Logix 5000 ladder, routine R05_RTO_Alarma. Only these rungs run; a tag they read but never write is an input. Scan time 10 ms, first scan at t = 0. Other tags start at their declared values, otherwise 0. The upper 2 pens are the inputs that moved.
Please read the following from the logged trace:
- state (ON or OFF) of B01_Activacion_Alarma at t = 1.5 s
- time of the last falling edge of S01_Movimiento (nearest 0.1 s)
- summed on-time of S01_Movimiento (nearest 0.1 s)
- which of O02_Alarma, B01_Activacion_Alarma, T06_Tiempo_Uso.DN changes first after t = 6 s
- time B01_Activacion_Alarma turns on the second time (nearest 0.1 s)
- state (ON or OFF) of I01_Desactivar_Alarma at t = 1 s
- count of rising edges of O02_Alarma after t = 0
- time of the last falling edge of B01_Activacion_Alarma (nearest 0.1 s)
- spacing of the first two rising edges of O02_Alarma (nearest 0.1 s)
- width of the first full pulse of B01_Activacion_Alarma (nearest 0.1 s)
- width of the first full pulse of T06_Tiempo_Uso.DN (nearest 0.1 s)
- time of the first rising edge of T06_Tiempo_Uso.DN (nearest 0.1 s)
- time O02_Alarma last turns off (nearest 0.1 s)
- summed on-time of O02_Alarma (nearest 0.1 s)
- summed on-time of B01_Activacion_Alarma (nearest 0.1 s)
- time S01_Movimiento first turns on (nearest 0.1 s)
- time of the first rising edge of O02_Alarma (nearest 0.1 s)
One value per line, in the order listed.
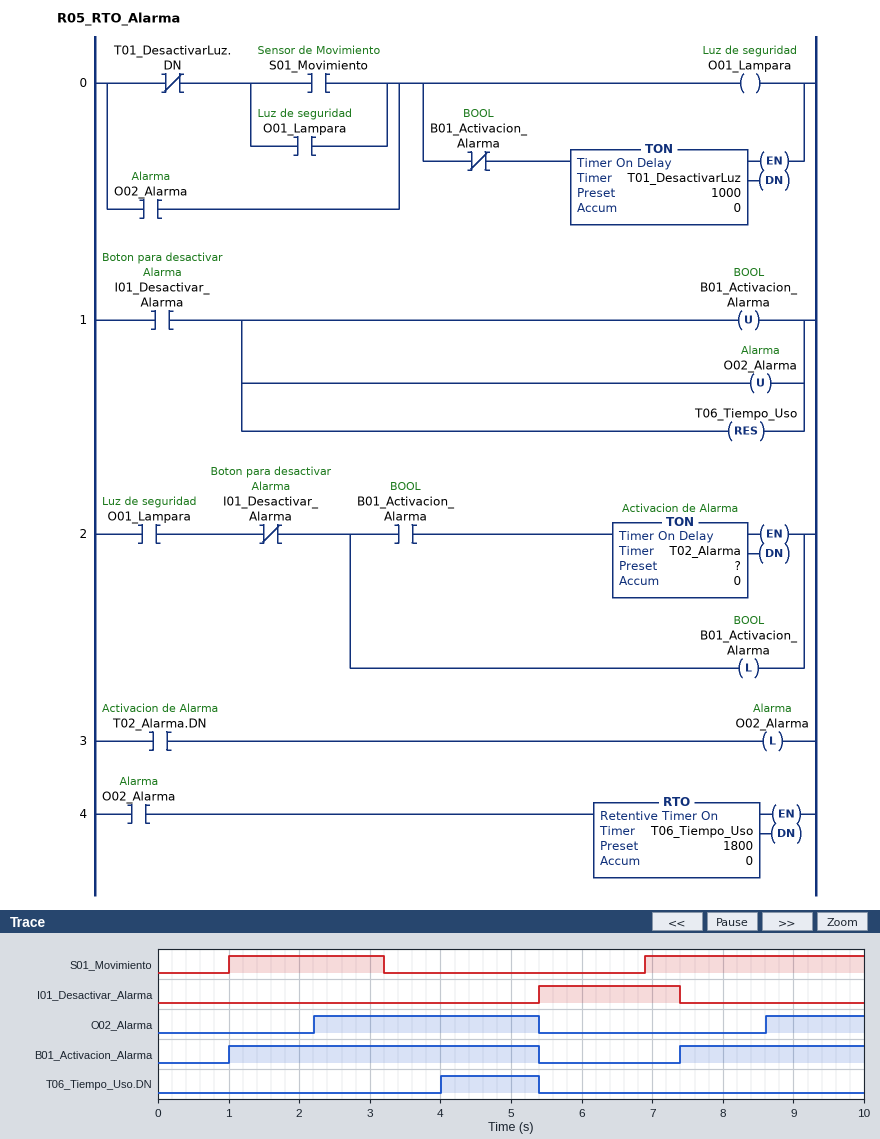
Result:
ON
3.2 s
5.3 s
B01_Activacion_Alarma
7.4 s
OFF
2
5.4 s
6.4 s
4.4 s
1.4 s
4.0 s
5.4 s
4.6 s
7.0 s
1.0 s
2.2 s
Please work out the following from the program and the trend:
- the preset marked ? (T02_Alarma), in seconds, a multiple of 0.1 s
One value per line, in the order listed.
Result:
1.2 s
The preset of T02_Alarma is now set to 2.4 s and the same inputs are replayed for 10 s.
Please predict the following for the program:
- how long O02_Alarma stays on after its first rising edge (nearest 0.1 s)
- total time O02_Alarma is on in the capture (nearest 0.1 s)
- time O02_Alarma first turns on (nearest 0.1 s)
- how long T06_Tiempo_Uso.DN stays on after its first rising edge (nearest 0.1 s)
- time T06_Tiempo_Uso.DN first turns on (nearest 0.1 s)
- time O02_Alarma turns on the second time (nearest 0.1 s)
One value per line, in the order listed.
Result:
2.0 s
2.2 s
3.4 s
0.2 s
5.2 s
9.8 s
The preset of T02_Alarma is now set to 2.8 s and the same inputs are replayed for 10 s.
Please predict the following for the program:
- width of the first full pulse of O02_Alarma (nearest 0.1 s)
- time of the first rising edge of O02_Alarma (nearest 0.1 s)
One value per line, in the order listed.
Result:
1.6 s
3.8 s
